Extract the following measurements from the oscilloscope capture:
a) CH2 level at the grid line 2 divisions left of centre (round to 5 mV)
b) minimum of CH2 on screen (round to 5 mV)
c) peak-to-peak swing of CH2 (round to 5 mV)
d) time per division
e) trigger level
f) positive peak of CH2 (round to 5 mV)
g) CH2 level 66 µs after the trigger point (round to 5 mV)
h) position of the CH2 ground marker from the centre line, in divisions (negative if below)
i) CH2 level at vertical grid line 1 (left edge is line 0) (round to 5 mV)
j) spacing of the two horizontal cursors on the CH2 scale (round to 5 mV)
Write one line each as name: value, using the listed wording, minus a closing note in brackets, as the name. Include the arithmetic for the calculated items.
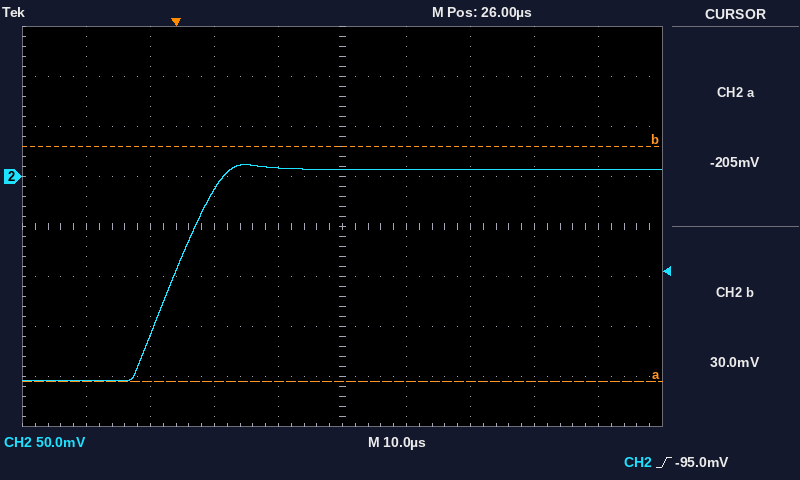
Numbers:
CH2 level at the grid line 2 divisions left of centre: -15 mV
minimum of CH2 on screen: -205 mV
peak-to-peak swing of CH2: 10 mV − (-205 mV) = 215 mV
time per division: 10 µs
trigger level: -95.0 mV
positive peak of CH2: 10 mV
CH2 level 66 µs after the trigger point: 5 mV
position of the CH2 ground marker from the centre line, in divisions: +1.0 div
CH2 level at vertical grid line 1 (left edge is line 0): -205 mV
spacing of the two horizontal cursors on the CH2 scale: 235 mV
